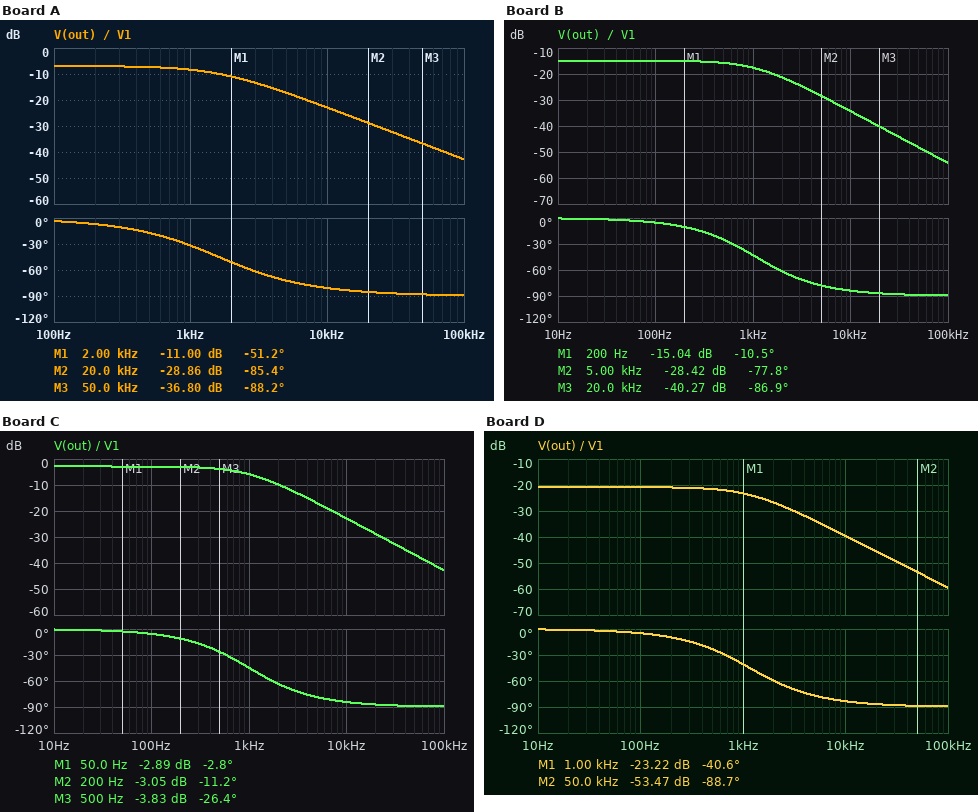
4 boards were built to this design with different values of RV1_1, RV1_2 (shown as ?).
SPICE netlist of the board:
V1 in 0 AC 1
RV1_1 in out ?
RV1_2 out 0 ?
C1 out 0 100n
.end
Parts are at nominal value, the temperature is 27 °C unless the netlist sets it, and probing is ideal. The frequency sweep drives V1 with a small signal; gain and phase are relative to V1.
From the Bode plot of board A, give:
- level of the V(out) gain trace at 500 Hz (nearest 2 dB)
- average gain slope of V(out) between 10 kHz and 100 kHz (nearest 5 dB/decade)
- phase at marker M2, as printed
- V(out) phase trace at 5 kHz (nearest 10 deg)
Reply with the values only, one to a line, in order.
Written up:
-8 dB
-20 dB/decade
-85.4 deg
-70 deg
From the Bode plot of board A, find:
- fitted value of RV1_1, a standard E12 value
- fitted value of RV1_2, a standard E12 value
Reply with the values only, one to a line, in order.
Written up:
2.2 kΩ
1.8 kΩ
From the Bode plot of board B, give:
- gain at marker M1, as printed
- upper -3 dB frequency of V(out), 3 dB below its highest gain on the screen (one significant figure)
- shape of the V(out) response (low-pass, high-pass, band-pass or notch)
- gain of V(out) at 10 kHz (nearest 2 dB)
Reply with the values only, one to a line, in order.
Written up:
-15.04 dB
1 kHz
low-pass
-34 dB
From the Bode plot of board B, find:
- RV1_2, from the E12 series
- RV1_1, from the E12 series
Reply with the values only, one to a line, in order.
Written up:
1.8 kΩ
8.2 kΩ
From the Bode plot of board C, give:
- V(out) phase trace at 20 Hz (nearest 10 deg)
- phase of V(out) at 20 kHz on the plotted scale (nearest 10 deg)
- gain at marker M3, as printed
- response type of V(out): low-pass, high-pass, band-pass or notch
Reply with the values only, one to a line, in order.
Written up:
0 deg
-90 deg
-3.83 dB
low-pass
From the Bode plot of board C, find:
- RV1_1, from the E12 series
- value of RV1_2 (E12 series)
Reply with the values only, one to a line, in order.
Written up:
2.2 kΩ
5.6 kΩ
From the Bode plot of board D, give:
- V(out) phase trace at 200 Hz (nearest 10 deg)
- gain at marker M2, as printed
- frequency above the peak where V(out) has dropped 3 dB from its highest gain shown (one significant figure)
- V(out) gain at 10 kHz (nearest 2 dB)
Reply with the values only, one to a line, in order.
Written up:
-10 deg
-53.47 dB
1 kHz
-40 dB
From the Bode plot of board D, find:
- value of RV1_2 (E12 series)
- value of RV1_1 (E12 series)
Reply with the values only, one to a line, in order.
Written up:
1.5 kΩ
15 kΩ
